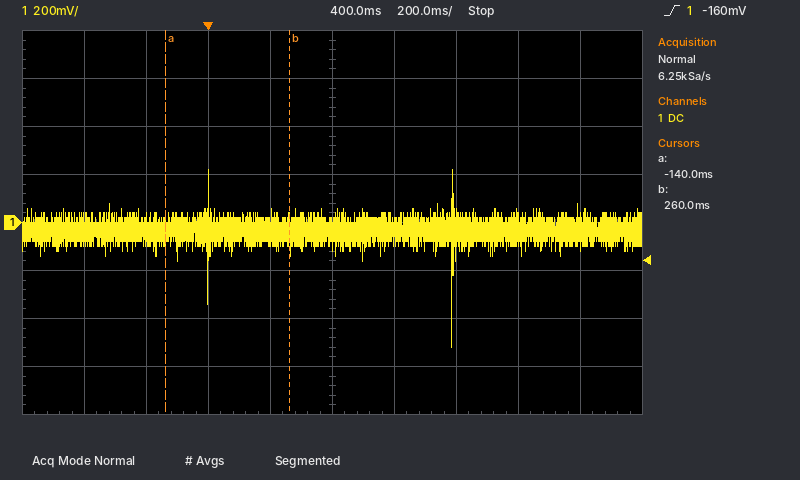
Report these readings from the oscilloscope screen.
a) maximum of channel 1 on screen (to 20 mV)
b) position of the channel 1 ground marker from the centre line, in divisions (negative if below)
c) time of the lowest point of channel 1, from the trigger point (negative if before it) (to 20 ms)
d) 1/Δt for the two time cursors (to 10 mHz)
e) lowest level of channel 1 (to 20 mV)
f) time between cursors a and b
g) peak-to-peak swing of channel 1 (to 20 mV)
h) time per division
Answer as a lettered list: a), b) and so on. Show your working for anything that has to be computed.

a) 220 mV
b) 0.0 div
c) +780 ms
d) 1 / 400 ms ≈ 2.50 Hz
e) -520 mV
f) 260 ms − (-140 ms) = 400 ms
g) 220 mV − (-520 mV) = 740 mV
h) 200 ms
